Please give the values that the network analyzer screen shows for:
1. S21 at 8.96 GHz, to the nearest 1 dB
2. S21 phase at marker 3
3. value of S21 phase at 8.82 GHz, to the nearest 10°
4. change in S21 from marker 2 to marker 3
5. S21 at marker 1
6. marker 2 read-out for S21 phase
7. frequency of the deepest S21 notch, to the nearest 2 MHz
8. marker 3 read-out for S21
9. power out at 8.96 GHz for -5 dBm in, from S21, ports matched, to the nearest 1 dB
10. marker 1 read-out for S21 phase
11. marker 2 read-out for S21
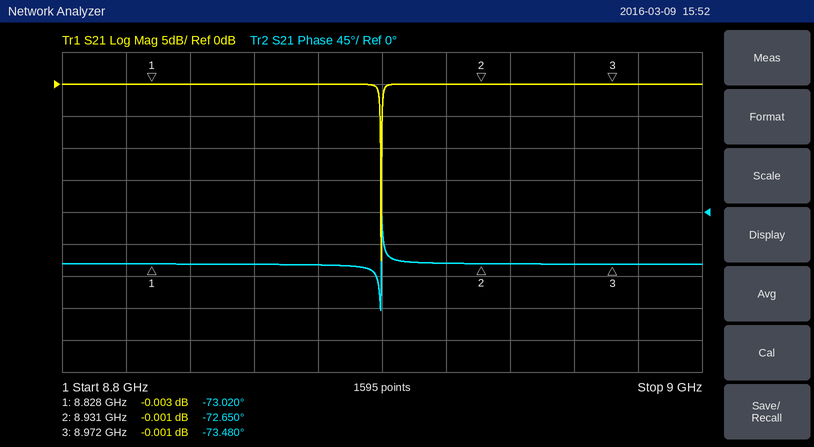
0 dB
-73.480°
-70°
0.000 dB
-0.003 dB
-72.650°
8.900 GHz
-0.001 dB
-5 dBm
-73.020°
-0.001 dB
